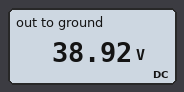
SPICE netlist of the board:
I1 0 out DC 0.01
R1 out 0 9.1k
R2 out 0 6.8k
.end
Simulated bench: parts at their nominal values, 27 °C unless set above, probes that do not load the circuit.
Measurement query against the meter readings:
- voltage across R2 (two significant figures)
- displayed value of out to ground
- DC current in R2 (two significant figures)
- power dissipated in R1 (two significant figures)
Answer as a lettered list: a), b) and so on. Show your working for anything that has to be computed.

a) 38.92 V = 39 V
b) 38.92 V
c) (38.92 V) / 6.8 kΩ = 5.7 mA
d) (38.92 V)^2 / 9.1 kΩ = 170 mW
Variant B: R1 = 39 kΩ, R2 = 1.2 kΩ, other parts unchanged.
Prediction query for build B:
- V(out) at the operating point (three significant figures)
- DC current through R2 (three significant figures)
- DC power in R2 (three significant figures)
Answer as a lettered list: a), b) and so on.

a) 11.6 V
b) 9.70 mA
c) 113 mW
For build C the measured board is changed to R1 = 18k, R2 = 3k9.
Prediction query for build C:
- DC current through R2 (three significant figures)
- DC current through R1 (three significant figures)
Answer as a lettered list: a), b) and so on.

a) 8.22 mA
b) 1.78 mA
